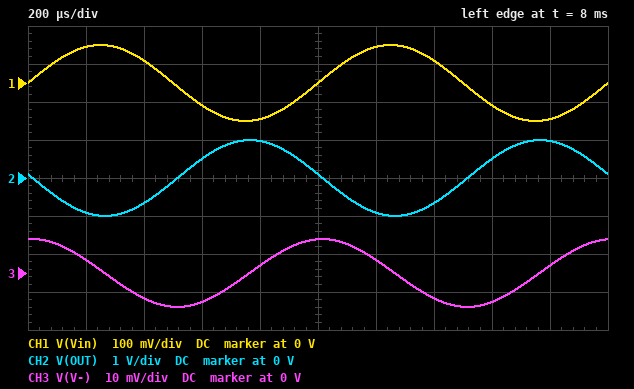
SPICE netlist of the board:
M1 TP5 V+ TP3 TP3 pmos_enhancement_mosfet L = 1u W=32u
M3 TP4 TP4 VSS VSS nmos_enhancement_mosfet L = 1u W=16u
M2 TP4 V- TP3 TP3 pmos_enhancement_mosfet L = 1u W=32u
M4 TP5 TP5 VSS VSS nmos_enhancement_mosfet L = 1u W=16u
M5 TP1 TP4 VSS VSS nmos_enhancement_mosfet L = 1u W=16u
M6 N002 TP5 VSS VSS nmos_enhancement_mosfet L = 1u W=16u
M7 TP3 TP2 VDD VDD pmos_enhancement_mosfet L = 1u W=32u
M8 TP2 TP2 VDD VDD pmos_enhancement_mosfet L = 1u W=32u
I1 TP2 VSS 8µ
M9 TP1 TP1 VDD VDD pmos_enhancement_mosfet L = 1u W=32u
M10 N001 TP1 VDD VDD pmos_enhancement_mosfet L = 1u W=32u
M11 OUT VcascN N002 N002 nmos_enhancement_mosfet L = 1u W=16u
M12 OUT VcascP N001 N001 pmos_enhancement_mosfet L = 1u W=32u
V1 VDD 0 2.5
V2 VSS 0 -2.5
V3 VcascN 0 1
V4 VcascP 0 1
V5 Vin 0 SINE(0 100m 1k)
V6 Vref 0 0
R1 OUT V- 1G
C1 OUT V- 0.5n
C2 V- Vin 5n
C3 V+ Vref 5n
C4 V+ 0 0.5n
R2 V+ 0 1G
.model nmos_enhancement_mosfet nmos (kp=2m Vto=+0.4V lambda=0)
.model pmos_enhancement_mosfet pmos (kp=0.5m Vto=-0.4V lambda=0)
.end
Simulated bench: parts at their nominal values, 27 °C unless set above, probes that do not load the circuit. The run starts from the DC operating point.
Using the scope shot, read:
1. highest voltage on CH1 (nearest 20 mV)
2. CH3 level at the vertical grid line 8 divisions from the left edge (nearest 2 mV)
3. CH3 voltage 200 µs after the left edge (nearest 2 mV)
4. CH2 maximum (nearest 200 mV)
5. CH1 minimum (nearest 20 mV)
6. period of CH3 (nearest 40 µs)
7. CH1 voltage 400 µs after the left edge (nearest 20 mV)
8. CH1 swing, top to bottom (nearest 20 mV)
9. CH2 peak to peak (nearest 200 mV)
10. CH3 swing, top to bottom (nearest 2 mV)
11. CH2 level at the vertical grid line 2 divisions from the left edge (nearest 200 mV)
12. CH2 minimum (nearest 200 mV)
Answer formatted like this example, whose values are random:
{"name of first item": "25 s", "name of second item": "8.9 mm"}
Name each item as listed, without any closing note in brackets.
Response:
{"highest voltage on CH1": "100 mV", "CH3 level at the vertical grid line 8 divisions from the left edge": "-8 mV", "CH3 voltage 200 µs after the left edge": "4 mV", "CH2 maximum": "1.0 V", "CH1 minimum": "-100 mV", "period of CH3": "1.00 ms", "CH1 voltage 400 µs after the left edge": "60 mV", "CH1 swing, top to bottom": "200 mV", "CH2 peak to peak": "2.0 V", "CH3 swing, top to bottom": "18 mV", "CH2 level at the vertical grid line 2 divisions from the left edge": "-600 mV", "CH2 minimum": "-1.0 V"}
